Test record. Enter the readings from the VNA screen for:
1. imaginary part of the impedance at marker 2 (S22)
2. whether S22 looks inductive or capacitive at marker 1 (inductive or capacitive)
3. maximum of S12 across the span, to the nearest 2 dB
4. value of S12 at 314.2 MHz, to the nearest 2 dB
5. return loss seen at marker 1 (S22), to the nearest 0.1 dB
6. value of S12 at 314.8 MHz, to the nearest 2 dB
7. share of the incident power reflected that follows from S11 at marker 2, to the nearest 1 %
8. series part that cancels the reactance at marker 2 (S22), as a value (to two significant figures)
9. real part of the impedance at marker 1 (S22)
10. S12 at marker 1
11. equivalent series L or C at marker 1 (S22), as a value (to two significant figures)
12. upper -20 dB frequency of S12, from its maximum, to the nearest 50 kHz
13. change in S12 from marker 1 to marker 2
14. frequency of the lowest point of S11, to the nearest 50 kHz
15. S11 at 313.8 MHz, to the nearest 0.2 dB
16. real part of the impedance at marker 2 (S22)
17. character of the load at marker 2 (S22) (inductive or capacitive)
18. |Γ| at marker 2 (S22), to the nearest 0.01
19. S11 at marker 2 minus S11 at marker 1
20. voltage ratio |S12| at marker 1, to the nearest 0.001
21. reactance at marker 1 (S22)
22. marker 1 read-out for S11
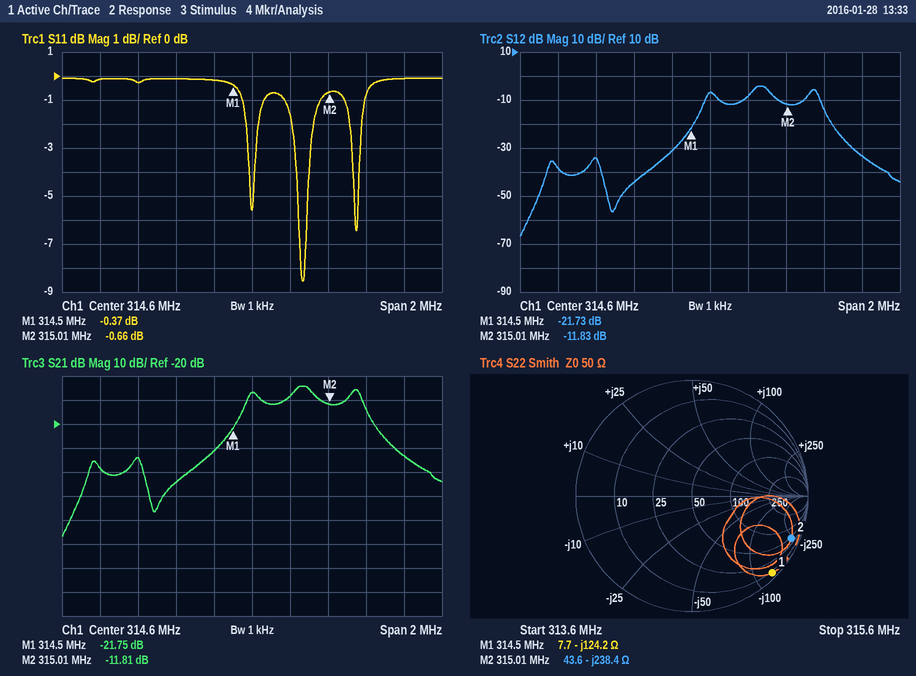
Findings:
-238.4 Ω
capacitive
-4 dB
-44 dB
0.4 dB
-8 dB
86 %
120 nH
7.7 Ω
-21.73 dB
4.1 pF
315.30 MHz
9.90 dB
314.85 MHz
-0.2 dB
43.6 Ω
capacitive
0.93
-0.29 dB
0.082
-124.2 Ω
-0.37 dB
